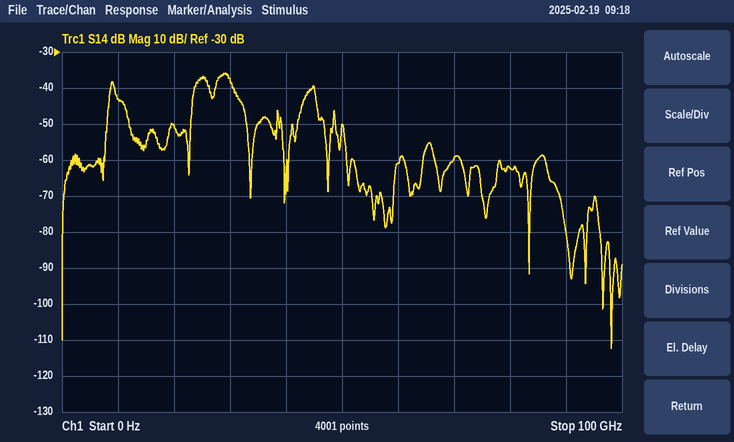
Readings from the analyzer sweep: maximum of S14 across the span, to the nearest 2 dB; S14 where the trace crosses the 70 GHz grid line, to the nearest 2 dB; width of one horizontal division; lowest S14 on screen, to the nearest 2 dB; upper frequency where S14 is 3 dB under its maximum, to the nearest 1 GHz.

-36 dB
-60 dB
10 GHz
-112 dB
30 GHz
